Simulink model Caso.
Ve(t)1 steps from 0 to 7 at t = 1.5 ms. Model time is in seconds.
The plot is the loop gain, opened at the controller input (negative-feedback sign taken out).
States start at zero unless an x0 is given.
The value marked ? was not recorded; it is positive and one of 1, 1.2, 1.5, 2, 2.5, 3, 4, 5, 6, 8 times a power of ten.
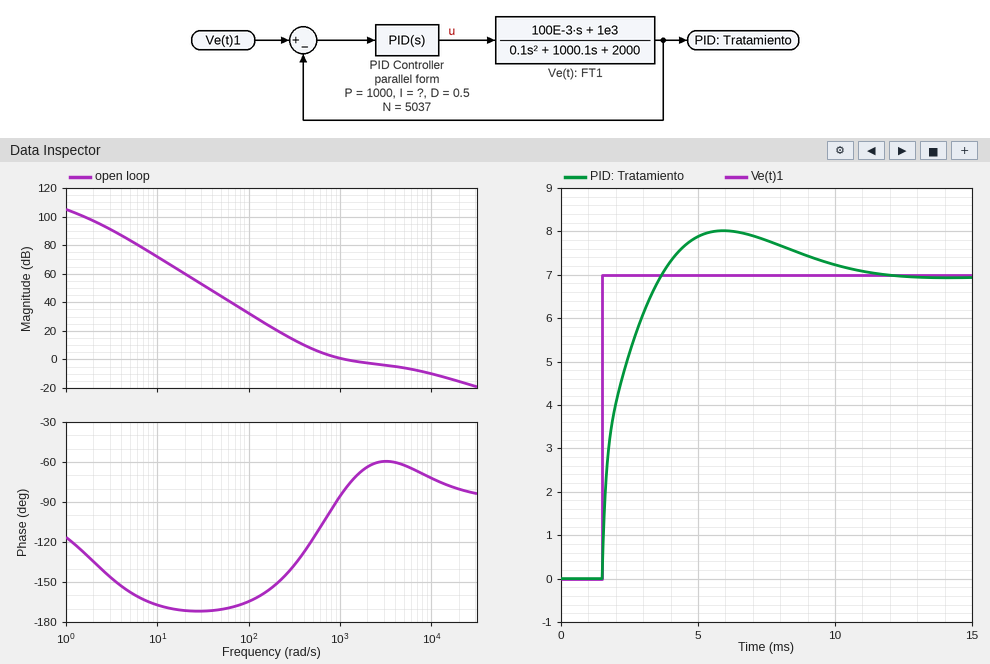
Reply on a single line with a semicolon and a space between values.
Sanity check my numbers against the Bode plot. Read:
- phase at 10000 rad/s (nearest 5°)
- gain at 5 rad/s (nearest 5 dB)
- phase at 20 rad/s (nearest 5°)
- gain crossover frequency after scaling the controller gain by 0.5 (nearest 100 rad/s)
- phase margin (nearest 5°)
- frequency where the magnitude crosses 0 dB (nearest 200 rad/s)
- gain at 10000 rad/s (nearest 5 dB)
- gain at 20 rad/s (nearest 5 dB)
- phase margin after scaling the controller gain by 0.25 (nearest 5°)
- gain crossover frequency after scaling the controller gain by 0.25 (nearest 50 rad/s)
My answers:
-70°; 85 dB; -170°; 600 rad/s; 100°; 1200 rad/s; -10 dB; 60 dB; 45°; 350 rad/s
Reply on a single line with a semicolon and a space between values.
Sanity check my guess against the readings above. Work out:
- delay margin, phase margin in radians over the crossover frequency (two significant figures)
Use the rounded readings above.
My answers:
0.0015 s
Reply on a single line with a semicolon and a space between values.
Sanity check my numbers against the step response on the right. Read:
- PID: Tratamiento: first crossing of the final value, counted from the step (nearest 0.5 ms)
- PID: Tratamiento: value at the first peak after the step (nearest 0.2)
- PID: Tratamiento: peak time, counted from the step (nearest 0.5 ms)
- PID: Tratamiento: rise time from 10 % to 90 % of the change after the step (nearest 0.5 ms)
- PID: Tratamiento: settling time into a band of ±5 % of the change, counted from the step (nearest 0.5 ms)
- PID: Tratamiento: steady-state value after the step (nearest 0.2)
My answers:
2.0 ms; 8.0; 4.5 ms; 1.5 ms; 8.0 ms; 7.0
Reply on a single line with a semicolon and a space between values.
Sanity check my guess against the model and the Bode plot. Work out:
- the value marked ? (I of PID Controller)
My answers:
400000
